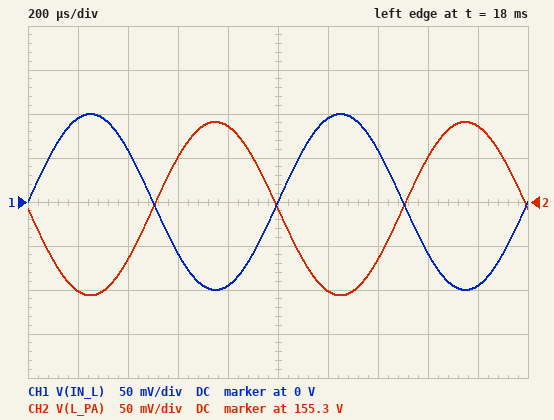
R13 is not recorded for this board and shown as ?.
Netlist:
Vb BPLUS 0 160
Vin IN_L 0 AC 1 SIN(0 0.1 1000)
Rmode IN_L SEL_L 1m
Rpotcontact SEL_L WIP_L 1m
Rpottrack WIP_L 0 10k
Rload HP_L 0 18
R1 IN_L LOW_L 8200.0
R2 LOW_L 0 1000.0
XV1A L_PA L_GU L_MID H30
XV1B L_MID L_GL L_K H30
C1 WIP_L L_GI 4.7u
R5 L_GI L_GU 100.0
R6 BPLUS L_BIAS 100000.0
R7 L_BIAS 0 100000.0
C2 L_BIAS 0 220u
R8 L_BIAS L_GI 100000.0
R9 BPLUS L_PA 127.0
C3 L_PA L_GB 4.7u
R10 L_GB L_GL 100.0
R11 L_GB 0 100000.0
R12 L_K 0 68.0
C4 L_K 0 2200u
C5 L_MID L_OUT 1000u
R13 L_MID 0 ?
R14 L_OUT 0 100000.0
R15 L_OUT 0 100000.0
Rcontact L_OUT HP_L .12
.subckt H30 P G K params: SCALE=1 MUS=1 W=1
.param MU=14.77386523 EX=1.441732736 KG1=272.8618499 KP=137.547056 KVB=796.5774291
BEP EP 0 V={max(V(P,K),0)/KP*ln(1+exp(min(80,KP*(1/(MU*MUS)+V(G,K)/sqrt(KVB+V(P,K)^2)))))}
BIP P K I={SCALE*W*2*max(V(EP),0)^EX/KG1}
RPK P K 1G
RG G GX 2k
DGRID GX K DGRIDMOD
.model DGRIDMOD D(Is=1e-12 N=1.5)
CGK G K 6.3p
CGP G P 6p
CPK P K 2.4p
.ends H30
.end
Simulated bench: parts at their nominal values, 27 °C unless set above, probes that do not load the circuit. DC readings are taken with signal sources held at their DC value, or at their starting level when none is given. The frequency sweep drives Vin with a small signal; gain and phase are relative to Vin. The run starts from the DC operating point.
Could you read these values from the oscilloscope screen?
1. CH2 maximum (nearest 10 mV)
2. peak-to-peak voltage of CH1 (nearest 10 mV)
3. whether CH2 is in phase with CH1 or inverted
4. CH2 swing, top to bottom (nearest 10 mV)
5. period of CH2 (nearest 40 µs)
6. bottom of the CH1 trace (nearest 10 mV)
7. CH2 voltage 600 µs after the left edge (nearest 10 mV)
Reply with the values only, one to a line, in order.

155.39 V
200 mV
inverted
200 mV
1.00 ms
-100 mV
155.35 V
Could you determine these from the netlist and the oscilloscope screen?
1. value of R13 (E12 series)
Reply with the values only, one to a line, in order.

150 kΩ
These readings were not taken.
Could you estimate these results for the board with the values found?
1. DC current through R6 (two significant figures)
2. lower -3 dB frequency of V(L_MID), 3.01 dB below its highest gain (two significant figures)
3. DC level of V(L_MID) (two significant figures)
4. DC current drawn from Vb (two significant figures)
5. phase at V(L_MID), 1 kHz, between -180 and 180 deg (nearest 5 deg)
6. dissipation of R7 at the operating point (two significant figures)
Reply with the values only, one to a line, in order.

800 µA
280 mHz
82 V
38 mA
0 deg
64 mW
